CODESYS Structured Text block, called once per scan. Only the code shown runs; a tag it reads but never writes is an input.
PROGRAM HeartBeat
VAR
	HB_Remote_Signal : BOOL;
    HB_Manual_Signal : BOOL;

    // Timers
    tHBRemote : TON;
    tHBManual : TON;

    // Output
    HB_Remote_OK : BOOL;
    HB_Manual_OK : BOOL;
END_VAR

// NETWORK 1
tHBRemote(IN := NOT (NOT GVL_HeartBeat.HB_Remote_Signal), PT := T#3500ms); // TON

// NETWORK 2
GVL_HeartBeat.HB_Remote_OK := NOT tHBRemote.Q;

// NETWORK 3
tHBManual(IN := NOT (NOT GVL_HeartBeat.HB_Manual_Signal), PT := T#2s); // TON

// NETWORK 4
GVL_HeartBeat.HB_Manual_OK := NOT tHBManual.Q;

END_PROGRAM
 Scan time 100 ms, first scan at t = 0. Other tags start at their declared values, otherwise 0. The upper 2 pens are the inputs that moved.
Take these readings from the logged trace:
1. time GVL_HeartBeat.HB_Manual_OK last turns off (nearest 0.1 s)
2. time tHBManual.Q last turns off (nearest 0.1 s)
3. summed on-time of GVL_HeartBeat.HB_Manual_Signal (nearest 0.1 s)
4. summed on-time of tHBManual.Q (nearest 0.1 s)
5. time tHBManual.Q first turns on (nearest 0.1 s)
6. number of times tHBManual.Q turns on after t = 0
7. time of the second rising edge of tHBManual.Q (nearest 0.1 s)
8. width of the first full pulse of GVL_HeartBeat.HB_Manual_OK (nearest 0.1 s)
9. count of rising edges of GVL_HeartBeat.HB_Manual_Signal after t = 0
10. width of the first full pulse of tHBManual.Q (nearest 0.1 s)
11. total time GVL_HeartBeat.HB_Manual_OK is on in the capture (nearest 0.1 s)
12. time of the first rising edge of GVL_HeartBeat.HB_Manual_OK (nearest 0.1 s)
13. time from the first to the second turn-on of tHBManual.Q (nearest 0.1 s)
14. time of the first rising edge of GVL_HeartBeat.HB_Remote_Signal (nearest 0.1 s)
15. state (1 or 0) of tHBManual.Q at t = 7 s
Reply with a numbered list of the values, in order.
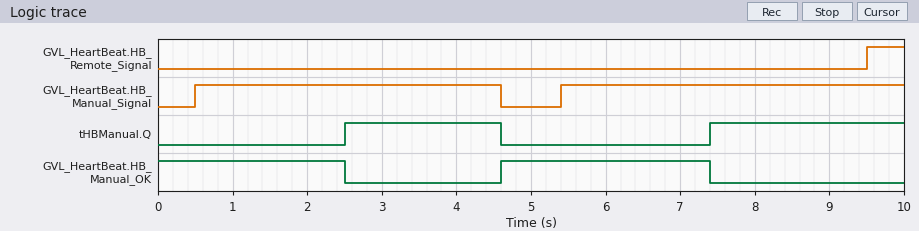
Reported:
1. 7.4 s
2. 4.6 s
3. 8.7 s
4. 4.7 s
5. 2.5 s
6. 2
7. 7.4 s
8. 2.8 s
9. 2
10. 2.1 s
11. 5.3 s
12. 4.6 s
13. 4.9 s
14. 9.5 s
15. 0
